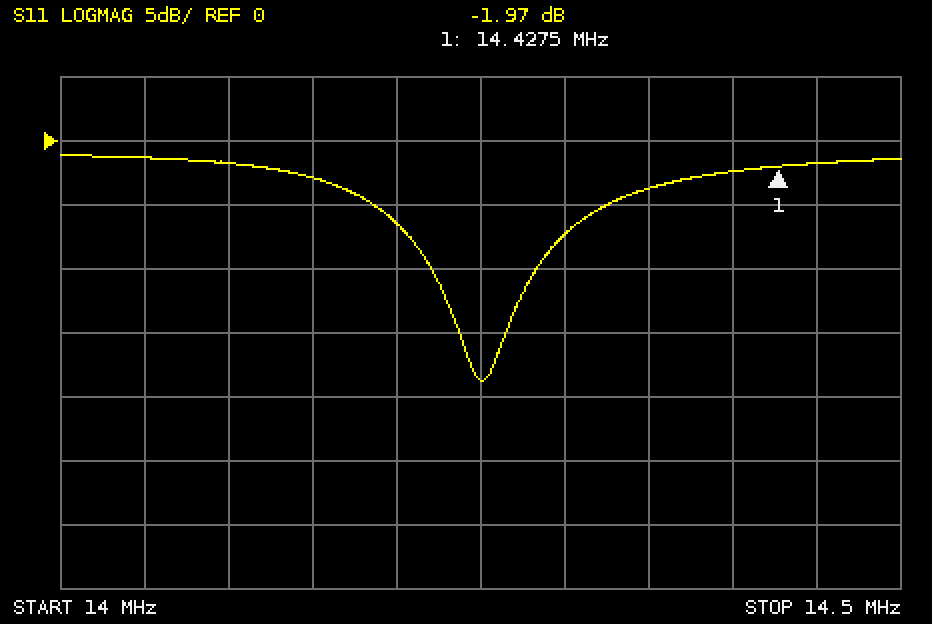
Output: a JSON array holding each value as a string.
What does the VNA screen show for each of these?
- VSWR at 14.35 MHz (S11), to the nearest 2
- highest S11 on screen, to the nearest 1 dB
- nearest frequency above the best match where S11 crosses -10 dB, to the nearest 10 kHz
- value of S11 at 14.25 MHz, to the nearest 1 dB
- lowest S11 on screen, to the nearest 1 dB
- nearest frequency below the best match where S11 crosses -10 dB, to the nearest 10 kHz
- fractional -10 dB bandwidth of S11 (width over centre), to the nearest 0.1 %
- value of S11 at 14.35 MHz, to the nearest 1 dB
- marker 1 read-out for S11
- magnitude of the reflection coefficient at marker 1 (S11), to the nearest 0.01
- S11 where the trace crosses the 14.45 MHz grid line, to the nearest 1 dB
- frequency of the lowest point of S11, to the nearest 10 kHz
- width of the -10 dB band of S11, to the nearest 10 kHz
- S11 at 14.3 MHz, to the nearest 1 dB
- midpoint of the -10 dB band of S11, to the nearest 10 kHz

["4", "-1 dB", "14.28 MHz", "-19 dB", "-19 dB", "14.22 MHz", "0.4 %", "-4 dB", "-1.97 dB", "0.80", "-2 dB", "14.25 MHz", "60 kHz", "-7 dB", "14.25 MHz"]
